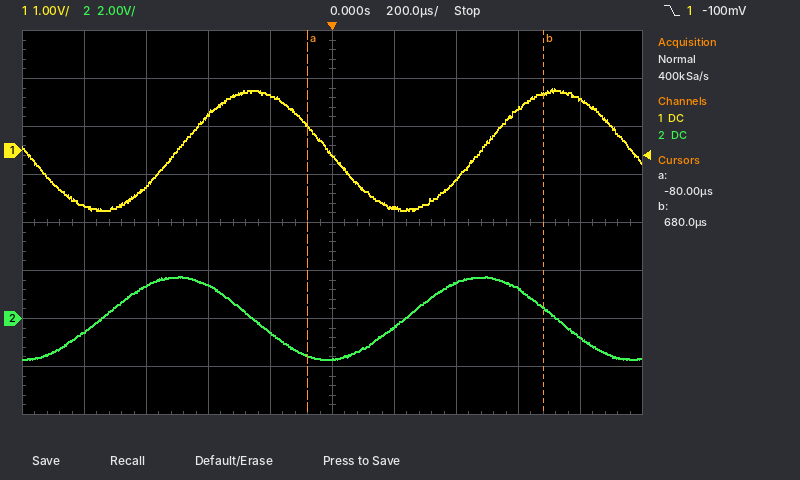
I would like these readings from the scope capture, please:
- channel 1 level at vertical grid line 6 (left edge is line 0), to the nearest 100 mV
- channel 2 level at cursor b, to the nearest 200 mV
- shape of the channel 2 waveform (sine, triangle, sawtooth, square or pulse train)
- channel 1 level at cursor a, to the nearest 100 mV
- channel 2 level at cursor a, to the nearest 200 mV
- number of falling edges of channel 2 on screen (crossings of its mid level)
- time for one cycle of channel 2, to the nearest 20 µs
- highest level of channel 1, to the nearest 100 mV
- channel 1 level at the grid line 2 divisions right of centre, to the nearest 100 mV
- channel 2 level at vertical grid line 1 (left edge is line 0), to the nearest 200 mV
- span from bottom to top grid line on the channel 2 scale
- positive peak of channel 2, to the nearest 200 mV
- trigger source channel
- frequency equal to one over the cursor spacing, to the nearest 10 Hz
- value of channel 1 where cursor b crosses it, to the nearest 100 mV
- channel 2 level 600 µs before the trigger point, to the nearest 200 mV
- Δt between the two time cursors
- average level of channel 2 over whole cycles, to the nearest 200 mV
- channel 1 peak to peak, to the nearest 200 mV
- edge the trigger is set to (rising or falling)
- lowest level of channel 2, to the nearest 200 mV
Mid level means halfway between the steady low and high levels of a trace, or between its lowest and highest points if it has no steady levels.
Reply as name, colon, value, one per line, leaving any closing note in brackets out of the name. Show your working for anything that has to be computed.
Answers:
channel 1 level at vertical grid line 6 (left edge is line 0), to the nearest 100 mV: -1.2 V
channel 2 level at cursor b, to the nearest 200 mV: 400 mV
shape of the channel 2 waveform: sine
channel 1 level at cursor a, to the nearest 100 mV: 500 mV
channel 2 level at cursor a, to the nearest 200 mV: -1.6 V
number of falling edges of channel 2 on screen: 2
time for one cycle of channel 2, to the nearest 20 µs: 980 µs
highest level of channel 1, to the nearest 100 mV: 1.3 V
channel 1 level at the grid line 2 divisions right of centre, to the nearest 100 mV: -600 mV
channel 2 level at vertical grid line 1 (left edge is line 0), to the nearest 200 mV: -600 mV
span from bottom to top grid line on the channel 2 scale: 16 V
positive peak of channel 2, to the nearest 200 mV: 1.8 V
trigger source channel: channel 1
frequency equal to one over the cursor spacing, to the nearest 10 Hz: 1 / 760 µs ≈ 1.32 kHz
value of channel 1 where cursor b crosses it, to the nearest 100 mV: 1.2 V
channel 2 level 600 µs before the trigger point, to the nearest 200 mV: 1.4 V
Δt between the two time cursors: 680 µs − (-80 µs) = 760 µs
average level of channel 2 over whole cycles, to the nearest 200 mV: (1.8 V + (-1.8 V)) / 2 ≈ 0.0 V
channel 1 peak to peak, to the nearest 200 mV: 2.6 V
edge the trigger is set to: falling
lowest level of channel 2, to the nearest 200 mV: -1.8 V
